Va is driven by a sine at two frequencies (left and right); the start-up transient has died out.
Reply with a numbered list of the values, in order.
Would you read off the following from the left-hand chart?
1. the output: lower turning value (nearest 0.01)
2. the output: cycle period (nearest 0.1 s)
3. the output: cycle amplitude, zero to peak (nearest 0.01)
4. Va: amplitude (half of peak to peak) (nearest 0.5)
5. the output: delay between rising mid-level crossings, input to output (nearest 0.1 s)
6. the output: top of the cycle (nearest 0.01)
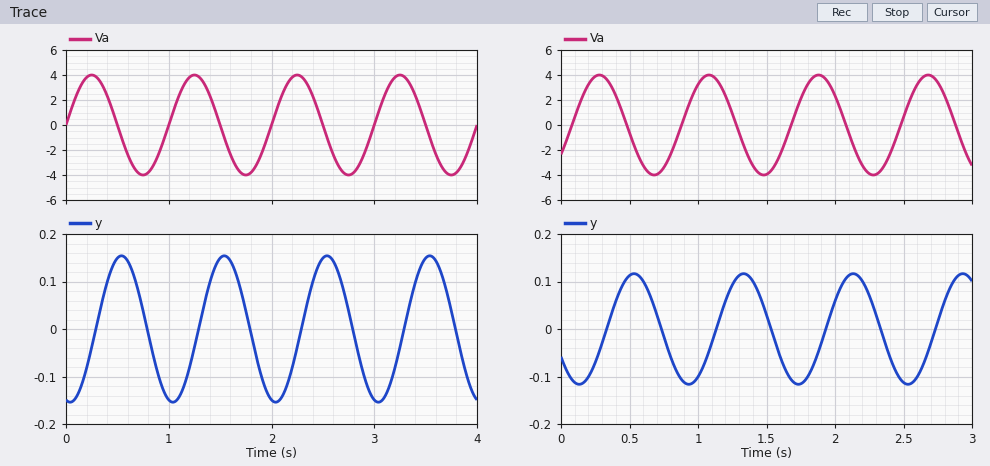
1. -0.15
2. 1.0 s
3. 0.15
4. 4.0
5. 0.3 s
6. 0.15
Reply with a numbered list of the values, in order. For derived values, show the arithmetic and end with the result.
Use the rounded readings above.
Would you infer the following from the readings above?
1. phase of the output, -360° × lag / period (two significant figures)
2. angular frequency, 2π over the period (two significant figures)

1. -360 × 0.3 / 1 = -110°
2. 2π / 1 = 6.3 rad/s
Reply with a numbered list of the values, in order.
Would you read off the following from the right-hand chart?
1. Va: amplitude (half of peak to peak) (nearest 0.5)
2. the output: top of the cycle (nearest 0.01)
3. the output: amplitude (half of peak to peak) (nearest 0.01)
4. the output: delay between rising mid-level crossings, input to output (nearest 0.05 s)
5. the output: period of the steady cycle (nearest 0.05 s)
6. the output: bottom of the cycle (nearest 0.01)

1. 4.0
2. 0.12
3. 0.12
4. 0.25 s
5. 0.80 s
6. -0.12
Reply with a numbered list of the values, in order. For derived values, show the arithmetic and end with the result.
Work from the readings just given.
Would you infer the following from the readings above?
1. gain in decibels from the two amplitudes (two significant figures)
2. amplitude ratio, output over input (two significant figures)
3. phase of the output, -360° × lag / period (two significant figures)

1. 20 log10(0.12 / 4) = -30 dB
2. 0.12 / 4 = 0.030
3. -360 × 0.25 / 0.8 = -110°
